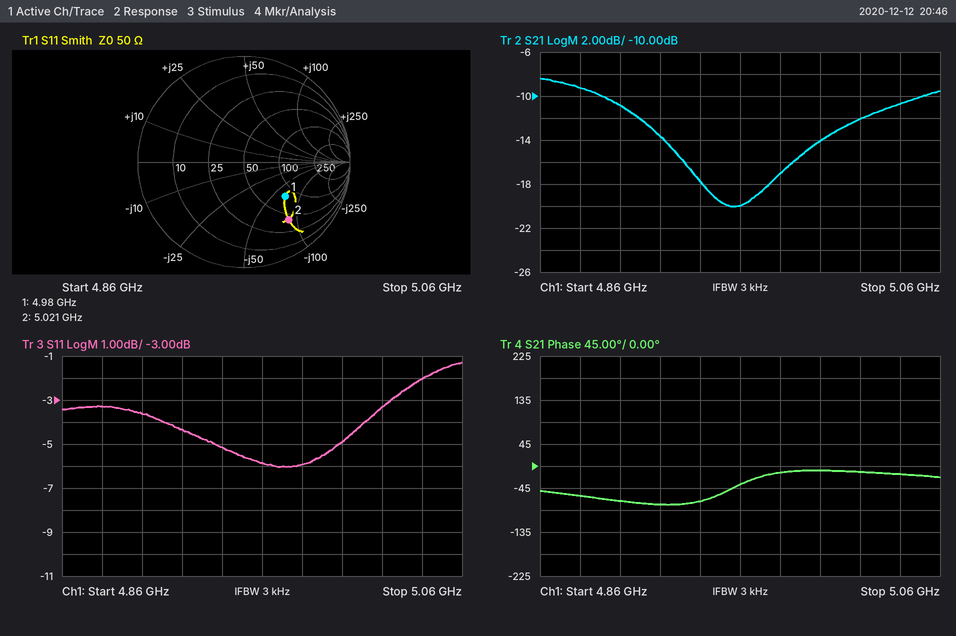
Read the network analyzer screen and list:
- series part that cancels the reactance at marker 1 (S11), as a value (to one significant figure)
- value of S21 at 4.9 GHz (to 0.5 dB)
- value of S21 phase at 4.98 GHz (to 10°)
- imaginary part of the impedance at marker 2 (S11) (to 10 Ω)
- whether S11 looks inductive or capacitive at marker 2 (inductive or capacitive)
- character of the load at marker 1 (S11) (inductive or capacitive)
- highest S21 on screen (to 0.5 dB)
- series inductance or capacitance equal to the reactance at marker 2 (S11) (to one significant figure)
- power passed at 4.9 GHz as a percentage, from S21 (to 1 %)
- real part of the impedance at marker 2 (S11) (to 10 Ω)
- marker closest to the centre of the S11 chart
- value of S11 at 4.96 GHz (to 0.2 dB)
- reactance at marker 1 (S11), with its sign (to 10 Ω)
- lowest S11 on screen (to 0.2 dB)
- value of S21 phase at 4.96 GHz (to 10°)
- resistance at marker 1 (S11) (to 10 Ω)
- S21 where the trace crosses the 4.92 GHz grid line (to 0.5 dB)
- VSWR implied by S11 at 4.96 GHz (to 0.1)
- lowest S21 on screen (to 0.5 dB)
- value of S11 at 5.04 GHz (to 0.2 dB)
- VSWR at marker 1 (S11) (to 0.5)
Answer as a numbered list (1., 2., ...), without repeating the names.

1. 2 nH
2. -11.0 dB
3. -10°
4. -90 Ω
5. capacitive
6. capacitive
7. -8.5 dB
8. 400 fF
9. 8 %
10. 40 Ω
11. marker 1
12. -5.8 dB
13. -70 Ω
14. -6.0 dB
15. -40°
16. 80 Ω
17. -13.5 dB
18. 3.1
19. -20.0 dB
20. -2.0 dB
21. 3.0
